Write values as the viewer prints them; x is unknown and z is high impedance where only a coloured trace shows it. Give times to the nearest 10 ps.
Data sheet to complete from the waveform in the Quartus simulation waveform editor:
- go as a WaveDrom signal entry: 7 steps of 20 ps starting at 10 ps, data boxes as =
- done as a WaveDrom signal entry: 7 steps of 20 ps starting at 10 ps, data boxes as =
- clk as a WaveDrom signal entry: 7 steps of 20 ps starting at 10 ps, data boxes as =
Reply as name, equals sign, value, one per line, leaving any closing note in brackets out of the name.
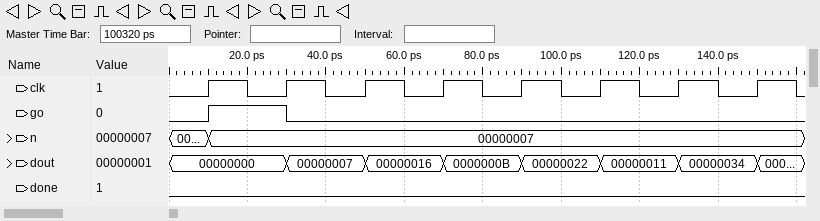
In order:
go as a WaveDrom signal entry: 7 steps of 20 ps starting at 10 ps, data boxes as = = {name: 'go', wave: '10.....'}
done as a WaveDrom signal entry: 7 steps of 20 ps starting at 10 ps, data boxes as = = {name: 'done', wave: '0......'}
clk as a WaveDrom signal entry: 7 steps of 20 ps starting at 10 ps, data boxes as = = {name: 'clk', wave: 'p......'}
